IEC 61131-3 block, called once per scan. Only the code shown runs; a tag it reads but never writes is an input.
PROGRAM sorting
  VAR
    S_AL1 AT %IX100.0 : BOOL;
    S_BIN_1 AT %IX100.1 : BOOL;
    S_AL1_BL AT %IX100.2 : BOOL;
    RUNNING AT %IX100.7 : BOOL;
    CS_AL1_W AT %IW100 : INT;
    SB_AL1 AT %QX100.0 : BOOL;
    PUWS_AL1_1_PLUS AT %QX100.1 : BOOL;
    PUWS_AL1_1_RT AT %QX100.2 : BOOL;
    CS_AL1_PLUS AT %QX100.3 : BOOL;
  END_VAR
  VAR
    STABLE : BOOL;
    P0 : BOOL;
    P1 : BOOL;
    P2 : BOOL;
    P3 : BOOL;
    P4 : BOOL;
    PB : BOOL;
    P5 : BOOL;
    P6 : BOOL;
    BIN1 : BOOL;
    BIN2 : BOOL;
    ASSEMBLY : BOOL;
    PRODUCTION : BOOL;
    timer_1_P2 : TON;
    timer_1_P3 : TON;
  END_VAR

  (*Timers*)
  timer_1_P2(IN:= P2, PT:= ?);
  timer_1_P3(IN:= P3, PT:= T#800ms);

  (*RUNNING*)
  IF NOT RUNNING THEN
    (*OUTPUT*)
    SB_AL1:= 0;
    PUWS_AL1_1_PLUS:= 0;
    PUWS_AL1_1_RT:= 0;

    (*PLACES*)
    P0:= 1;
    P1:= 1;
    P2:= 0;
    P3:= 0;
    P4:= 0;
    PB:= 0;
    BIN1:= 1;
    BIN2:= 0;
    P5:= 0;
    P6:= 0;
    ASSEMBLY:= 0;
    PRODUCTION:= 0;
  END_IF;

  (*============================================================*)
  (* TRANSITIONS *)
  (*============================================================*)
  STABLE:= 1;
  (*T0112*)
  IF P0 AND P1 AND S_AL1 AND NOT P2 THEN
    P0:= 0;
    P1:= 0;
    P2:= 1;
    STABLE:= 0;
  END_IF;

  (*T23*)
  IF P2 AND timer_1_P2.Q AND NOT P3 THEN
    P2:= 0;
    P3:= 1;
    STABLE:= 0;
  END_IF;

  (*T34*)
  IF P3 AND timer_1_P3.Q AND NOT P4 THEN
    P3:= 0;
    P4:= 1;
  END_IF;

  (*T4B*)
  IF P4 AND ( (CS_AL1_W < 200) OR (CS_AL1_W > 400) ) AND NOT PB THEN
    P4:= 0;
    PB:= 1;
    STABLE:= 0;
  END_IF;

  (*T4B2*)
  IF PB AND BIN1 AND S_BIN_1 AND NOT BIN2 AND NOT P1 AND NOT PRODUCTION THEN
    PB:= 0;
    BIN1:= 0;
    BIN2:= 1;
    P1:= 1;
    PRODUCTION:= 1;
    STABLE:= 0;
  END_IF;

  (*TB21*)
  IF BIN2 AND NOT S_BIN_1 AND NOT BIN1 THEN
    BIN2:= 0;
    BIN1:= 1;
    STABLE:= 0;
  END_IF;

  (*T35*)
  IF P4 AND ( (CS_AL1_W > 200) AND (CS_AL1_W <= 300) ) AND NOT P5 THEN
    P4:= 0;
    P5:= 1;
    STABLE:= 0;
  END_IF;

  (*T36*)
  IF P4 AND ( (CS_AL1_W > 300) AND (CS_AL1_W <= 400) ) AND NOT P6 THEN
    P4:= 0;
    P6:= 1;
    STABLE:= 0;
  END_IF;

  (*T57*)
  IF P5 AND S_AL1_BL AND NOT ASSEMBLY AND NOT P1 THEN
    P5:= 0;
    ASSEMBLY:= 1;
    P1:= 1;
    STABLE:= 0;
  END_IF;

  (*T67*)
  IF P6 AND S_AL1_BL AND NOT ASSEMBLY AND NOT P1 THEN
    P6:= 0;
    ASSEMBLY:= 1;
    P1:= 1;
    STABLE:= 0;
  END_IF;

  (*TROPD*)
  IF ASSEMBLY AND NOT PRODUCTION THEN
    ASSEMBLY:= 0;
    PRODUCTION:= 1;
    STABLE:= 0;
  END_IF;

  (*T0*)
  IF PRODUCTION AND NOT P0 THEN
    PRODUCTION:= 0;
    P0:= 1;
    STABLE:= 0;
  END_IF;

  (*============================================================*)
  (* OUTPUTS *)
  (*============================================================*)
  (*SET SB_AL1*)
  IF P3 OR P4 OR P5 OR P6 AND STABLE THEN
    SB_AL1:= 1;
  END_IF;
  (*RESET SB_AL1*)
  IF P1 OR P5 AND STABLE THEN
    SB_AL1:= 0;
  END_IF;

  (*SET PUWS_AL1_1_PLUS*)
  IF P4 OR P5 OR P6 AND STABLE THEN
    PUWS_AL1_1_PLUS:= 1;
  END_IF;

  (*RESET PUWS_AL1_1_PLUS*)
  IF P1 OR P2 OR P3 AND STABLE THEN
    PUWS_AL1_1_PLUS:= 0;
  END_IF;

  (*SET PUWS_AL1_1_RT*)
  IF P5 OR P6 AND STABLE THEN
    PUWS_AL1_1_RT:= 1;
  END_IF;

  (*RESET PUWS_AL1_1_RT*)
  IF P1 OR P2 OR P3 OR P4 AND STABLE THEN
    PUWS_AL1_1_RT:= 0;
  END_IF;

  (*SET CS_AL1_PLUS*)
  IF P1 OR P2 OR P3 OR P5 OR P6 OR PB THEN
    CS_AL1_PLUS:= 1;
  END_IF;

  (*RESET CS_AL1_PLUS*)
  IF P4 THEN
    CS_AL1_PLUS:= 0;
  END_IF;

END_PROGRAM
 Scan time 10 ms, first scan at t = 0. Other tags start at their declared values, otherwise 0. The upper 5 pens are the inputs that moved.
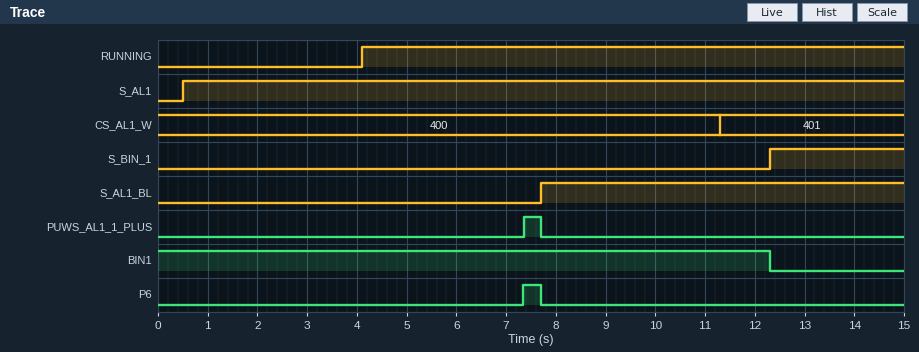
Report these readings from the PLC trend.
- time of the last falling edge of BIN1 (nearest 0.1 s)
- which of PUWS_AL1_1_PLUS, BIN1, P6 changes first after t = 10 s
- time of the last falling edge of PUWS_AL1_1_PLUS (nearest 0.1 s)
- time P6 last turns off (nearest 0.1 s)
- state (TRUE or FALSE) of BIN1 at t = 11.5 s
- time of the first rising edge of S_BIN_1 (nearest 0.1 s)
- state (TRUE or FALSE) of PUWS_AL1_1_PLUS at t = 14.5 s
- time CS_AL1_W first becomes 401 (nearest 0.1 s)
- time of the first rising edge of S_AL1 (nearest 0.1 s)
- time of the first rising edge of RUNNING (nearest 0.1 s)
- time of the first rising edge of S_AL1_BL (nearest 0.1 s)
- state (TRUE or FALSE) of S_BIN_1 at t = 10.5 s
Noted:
12.3 s
BIN1
7.7 s
7.7 s
TRUE
12.3 s
FALSE
11.3 s
0.5 s
4.1 s
7.7 s
FALSE
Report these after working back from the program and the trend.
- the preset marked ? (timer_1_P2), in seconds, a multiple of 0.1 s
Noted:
3.0 s
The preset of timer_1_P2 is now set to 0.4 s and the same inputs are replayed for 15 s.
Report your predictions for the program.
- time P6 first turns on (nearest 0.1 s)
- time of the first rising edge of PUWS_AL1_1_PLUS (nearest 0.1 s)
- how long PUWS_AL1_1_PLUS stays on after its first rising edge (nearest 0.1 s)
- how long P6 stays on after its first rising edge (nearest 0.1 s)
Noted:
5.1 s
5.1 s
2.6 s
2.6 s
